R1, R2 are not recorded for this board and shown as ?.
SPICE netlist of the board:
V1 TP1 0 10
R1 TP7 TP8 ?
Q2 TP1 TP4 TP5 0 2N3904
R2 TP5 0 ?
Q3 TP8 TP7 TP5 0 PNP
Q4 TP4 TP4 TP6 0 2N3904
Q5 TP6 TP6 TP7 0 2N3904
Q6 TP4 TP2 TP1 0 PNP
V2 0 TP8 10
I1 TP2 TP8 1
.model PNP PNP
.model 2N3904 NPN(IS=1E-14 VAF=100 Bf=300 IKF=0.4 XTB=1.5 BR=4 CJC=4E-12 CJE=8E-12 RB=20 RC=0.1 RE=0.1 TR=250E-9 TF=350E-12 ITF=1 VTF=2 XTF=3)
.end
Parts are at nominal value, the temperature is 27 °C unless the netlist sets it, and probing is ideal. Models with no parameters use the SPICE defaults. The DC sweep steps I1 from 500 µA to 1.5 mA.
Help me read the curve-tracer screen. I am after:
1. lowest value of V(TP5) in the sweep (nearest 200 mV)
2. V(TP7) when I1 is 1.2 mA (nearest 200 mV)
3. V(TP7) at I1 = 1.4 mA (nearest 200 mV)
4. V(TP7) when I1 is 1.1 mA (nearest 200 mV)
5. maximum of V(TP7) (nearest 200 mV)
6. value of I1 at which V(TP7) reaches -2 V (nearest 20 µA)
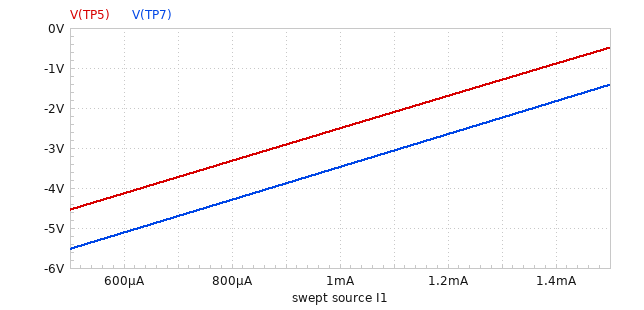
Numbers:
-4.6 V
-2.6 V
-1.8 V
-3.0 V
-1.4 V
1.36 mA
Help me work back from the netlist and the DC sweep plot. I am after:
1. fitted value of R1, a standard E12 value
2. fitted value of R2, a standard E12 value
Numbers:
56 Ω
1.5 Ω
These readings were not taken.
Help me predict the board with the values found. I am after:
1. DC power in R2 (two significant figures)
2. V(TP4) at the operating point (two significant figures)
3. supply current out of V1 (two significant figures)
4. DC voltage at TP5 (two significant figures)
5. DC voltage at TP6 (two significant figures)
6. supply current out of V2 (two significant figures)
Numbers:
24 W
10 V
5.3 A
6.0 V
9.1 V
1.3 A
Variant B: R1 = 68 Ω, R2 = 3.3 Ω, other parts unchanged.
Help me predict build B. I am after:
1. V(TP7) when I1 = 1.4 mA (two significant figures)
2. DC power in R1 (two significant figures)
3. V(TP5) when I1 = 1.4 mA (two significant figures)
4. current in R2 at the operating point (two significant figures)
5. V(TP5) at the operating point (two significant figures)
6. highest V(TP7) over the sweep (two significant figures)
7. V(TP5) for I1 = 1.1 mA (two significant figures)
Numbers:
-500 mV
4.9 W
330 mV
2.4 A
7.8 V
110 mV
-1.3 V
